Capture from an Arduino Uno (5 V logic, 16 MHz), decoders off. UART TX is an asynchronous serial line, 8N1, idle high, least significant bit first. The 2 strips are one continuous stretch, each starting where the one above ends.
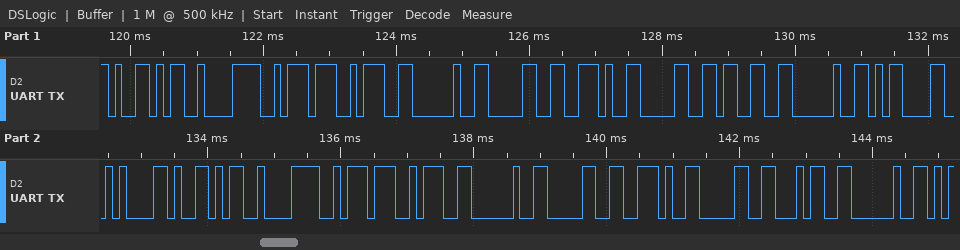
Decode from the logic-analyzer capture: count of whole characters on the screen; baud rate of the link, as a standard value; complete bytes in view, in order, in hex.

22
9600 baud
59 C2 BA 3A 20 30 2E 30 33 20 0D 0A 59 C2 BA 3A 20 30 2E 30 34 20
